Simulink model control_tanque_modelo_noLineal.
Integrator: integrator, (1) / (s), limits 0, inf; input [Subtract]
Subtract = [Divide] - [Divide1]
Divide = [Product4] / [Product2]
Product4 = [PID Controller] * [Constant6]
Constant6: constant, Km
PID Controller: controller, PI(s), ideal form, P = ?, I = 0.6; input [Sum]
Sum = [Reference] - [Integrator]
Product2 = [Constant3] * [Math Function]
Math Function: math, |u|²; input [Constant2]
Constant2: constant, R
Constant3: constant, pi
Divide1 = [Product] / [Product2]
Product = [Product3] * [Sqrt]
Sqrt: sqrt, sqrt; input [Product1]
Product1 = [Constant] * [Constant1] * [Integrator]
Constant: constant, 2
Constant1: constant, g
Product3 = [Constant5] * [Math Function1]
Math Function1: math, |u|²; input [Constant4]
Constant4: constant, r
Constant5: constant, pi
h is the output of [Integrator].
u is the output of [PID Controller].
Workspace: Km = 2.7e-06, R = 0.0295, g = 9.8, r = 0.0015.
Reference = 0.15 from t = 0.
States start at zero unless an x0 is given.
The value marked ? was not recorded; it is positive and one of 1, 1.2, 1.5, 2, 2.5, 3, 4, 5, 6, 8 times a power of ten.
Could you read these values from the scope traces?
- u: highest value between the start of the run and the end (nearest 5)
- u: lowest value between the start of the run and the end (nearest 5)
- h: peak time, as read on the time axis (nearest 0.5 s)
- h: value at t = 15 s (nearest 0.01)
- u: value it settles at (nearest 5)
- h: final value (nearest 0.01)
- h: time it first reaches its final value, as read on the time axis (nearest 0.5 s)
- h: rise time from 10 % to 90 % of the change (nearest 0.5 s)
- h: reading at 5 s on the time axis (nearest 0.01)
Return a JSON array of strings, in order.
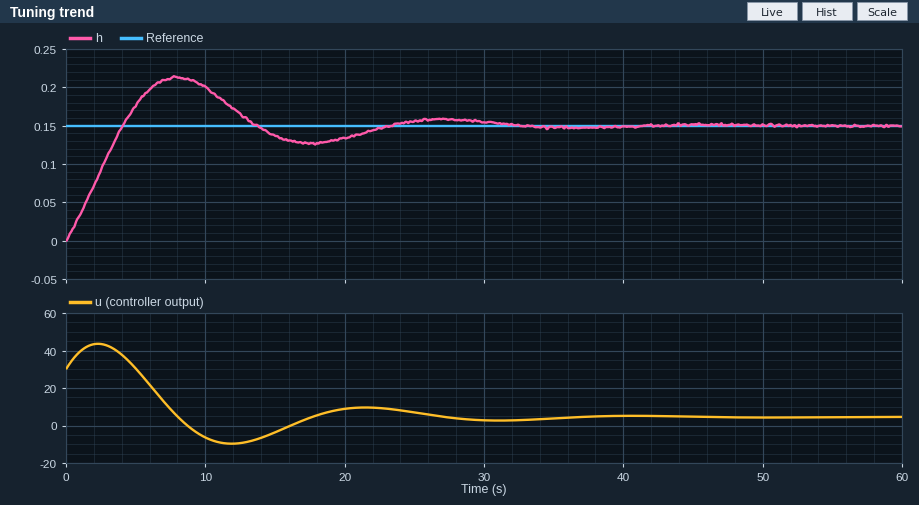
["45", "-10", "8.0 s", "0.14", "5", "0.15", "4.0 s", "3.0 s", "0.18"]
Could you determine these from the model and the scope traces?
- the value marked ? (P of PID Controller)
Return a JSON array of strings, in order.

["200"]
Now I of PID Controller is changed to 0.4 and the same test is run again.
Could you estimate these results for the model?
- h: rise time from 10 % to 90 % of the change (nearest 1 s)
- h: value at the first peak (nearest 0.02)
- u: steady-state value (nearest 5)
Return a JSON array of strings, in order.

["4 s", "0.20", "5"]
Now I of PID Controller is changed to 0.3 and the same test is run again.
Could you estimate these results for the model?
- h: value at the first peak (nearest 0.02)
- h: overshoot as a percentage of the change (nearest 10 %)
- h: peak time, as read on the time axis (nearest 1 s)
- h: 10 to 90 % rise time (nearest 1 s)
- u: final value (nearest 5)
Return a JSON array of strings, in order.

["0.20", "30 %", "11 s", "4 s", "5"]
